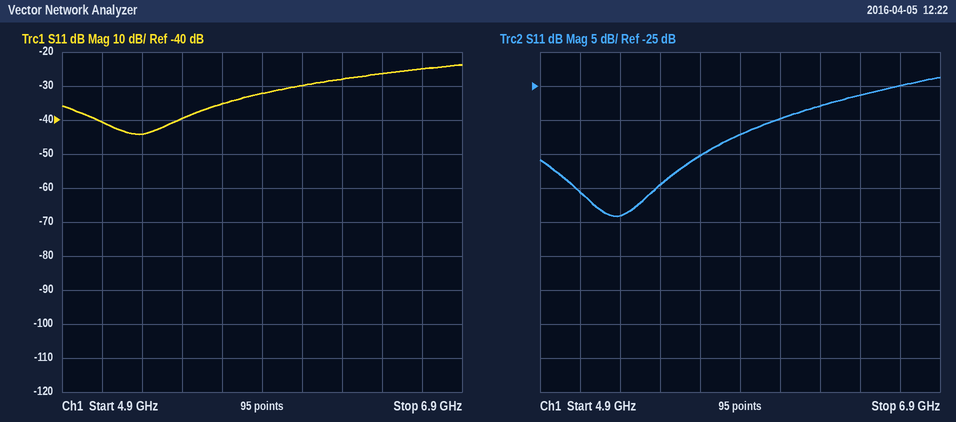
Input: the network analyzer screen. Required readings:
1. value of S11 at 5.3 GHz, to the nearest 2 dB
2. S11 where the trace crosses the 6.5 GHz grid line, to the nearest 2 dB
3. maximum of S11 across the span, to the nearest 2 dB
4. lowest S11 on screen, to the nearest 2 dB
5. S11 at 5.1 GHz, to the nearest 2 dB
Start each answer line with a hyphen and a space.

- -44 dB
- -26 dB
- -24 dB
- -44 dB
- -40 dB
